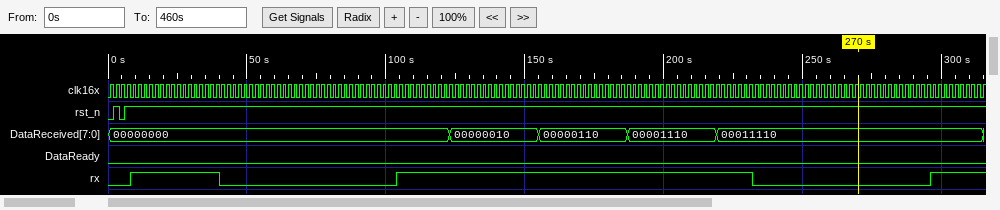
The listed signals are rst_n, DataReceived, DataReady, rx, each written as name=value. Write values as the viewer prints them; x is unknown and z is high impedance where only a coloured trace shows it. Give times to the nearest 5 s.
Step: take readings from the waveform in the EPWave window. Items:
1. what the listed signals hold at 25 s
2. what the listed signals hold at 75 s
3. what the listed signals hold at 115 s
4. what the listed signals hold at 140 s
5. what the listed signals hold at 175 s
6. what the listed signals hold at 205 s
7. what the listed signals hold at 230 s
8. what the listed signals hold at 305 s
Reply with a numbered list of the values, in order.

1. rst_n=1, DataReceived=00000000, DataReady=0, rx=1
2. rst_n=1, DataReceived=00000000, DataReady=0, rx=0
3. rst_n=1, DataReceived=00000000, DataReady=0, rx=1
4. rst_n=1, DataReceived=00000010, DataReady=0, rx=1
5. rst_n=1, DataReceived=00000110, DataReady=0, rx=1
6. rst_n=1, DataReceived=00001110, DataReady=0, rx=1
7. rst_n=1, DataReceived=00011110, DataReady=0, rx=1
8. rst_n=1, DataReceived=00011110, DataReady=0, rx=1
